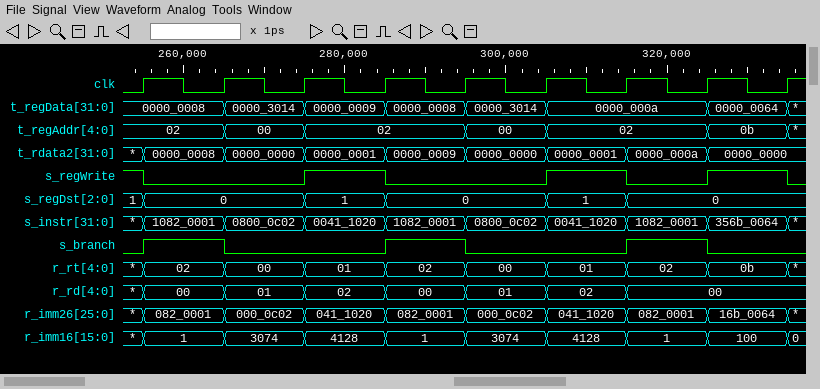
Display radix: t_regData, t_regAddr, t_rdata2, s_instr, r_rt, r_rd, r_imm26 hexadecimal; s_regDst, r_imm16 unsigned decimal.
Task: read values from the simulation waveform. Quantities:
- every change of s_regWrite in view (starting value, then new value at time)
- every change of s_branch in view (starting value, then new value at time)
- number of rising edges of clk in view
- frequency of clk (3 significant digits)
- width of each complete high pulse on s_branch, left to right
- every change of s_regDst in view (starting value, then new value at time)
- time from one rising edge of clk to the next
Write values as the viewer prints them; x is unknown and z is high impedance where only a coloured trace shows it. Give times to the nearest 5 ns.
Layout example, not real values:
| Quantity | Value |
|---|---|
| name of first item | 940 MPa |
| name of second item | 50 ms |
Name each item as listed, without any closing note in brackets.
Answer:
| Quantity | Value |
|---|---|
| every change of s_regWrite in view | 1, 0 at 255 ns, 1 at 275 ns, 0 at 285 ns, 1 at 305 ns, 0 at 315 ns, 1 at 325 ns, 0 at 335 ns |
| every change of s_branch in view | 0, 1 at 255 ns, 0 at 265 ns, 1 at 285 ns, 0 at 295 ns, 1 at 315 ns, 0 at 325 ns |
| number of rising edges of clk in view | 9 |
| frequency of clk | 100 MHz |
| width of each complete high pulse on s_branch, left to right | 10 ns, 10 ns, 10 ns |
| every change of s_regDst in view | 1, 0 at 255 ns, 1 at 275 ns, 0 at 285 ns, 1 at 305 ns, 0 at 315 ns |
| time from one rising edge of clk to the next | 10 ns |
